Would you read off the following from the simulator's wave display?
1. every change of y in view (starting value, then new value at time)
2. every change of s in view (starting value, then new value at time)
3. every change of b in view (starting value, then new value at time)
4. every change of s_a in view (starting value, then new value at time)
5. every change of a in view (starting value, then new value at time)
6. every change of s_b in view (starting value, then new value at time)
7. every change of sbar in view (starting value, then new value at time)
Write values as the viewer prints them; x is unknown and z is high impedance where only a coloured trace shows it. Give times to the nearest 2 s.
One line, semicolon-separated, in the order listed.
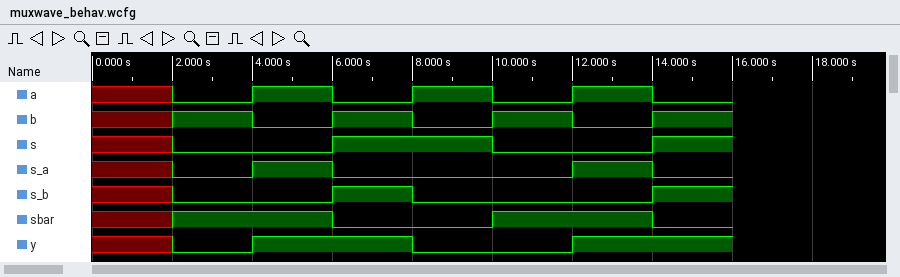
x, 0 at 2 s, 1 at 4 s, 0 at 8 s, 1 at 12 s; x, 0 at 2 s, 1 at 6 s, 0 at 10 s, 1 at 14 s; x, 1 at 2 s, 0 at 4 s, 1 at 6 s, 0 at 8 s, 1 at 10 s, 0 at 12 s, 1 at 14 s; x, 0 at 2 s, 1 at 4 s, 0 at 6 s, 1 at 12 s, 0 at 14 s; x, 0 at 2 s, 1 at 4 s, 0 at 6 s, 1 at 8 s, 0 at 10 s, 1 at 12 s, 0 at 14 s; x, 0 at 2 s, 1 at 6 s, 0 at 8 s, 1 at 14 s; x, 1 at 2 s, 0 at 6 s, 1 at 10 s, 0 at 14 s
